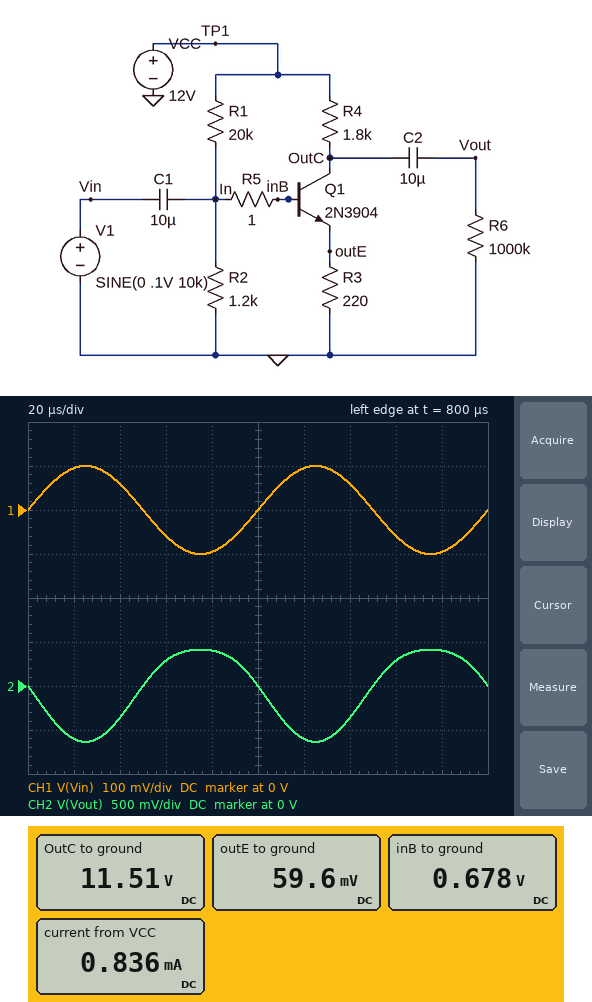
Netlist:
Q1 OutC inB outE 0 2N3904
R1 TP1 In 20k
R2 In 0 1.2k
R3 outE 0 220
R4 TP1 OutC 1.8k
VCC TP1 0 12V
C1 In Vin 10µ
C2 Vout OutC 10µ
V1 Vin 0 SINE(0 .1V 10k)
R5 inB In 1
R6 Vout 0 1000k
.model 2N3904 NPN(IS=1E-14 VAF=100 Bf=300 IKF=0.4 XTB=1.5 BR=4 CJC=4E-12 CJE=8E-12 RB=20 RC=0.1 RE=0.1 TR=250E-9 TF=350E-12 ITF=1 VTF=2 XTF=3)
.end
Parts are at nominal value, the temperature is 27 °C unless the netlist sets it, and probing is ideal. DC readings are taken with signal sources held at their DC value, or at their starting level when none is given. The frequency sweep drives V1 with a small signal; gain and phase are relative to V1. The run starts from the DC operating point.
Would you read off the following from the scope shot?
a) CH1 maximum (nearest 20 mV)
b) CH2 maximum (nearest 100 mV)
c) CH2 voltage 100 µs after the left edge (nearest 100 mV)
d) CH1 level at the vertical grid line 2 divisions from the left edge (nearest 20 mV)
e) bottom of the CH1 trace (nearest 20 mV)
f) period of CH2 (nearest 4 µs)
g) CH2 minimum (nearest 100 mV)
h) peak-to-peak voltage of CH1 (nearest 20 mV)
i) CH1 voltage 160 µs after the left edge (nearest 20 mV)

100 mV
400 mV
0 V
60 mV
-100 mV
100 µs
-600 mV
200 mV
-60 mV
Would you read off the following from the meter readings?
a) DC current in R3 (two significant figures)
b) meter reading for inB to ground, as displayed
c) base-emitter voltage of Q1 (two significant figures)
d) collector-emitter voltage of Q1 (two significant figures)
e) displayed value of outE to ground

270 µA
0.678 V
620 mV
11 V
59.6 mV
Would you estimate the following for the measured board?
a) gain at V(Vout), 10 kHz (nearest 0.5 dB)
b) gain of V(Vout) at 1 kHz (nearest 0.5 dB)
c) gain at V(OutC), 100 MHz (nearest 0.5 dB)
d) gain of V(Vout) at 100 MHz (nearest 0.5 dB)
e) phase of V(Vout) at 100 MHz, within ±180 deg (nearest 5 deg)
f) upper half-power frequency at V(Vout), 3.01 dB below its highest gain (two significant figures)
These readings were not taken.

15.0 dB
15.0 dB
8.5 dB
8.5 dB
70 deg
50 MHz
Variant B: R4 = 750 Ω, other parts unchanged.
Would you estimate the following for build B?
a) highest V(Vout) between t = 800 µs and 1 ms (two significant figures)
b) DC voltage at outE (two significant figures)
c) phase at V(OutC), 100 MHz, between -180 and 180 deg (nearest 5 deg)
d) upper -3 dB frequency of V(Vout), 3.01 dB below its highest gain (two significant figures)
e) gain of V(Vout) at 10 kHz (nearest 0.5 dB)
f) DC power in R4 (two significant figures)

170 mV
60 mV
90 deg
130 MHz
7.5 dB
55 µW
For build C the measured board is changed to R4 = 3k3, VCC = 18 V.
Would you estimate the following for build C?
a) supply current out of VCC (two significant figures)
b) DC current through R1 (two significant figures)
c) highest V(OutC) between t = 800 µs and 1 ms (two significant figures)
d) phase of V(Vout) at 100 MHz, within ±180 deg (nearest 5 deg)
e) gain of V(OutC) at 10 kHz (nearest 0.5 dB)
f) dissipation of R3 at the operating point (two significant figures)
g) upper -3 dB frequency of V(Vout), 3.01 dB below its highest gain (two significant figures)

2.4 mA
850 µA
14 V
75 deg
23.0 dB
550 µW
28 MHz
